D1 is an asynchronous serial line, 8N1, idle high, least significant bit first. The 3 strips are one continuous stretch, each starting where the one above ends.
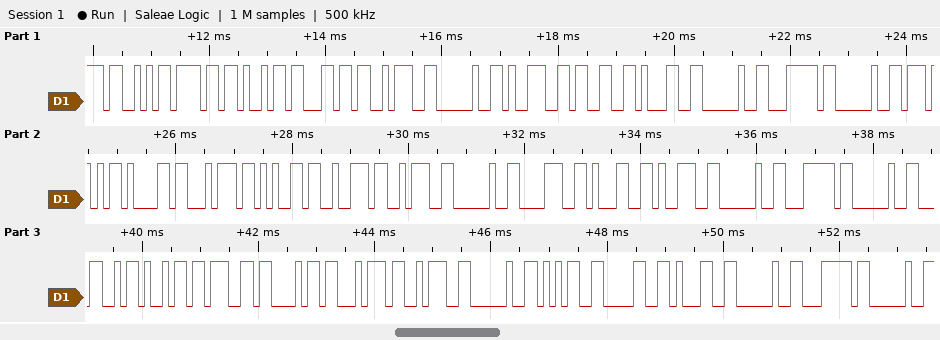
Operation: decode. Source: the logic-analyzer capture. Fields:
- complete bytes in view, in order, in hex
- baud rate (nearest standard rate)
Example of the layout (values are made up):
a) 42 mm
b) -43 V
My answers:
a) 53 6F 69 6C 3A 20 39 33 31 20 7C 20 57 61 74 65 72 3A 20 38 31 39 20 7C 20 4C 69 67 68 74 3A 20 35 30 31 20 7C 20
b) 9600 baud
